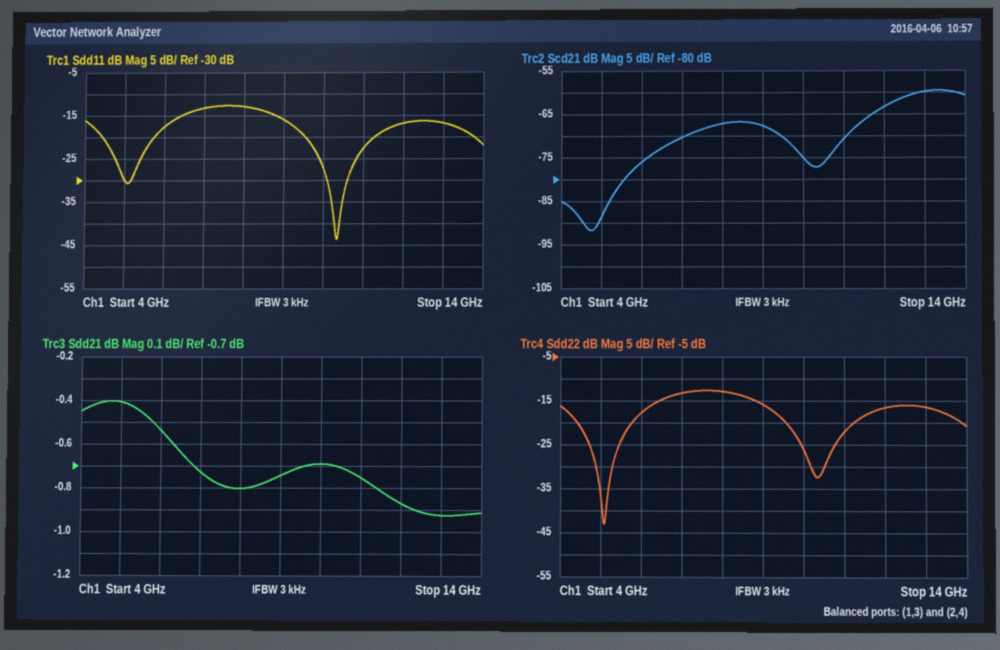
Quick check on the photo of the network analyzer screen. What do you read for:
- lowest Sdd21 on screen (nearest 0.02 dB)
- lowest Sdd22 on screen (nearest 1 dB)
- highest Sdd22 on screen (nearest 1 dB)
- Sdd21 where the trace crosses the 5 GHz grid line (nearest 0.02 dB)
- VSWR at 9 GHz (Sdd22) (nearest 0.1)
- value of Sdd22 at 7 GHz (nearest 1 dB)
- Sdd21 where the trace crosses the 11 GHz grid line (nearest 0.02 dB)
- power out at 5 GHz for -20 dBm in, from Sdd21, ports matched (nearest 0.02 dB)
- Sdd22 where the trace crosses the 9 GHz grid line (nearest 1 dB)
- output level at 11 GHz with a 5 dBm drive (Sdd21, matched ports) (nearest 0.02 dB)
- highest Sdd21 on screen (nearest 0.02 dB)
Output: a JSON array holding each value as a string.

["-0.92 dB", "-43 dB", "-13 dB", "-0.40 dB", "1.4", "-13 dB", "-0.76 dB", "-20.40 dBm", "-16 dB", "4.24 dBm", "-0.40 dB"]
